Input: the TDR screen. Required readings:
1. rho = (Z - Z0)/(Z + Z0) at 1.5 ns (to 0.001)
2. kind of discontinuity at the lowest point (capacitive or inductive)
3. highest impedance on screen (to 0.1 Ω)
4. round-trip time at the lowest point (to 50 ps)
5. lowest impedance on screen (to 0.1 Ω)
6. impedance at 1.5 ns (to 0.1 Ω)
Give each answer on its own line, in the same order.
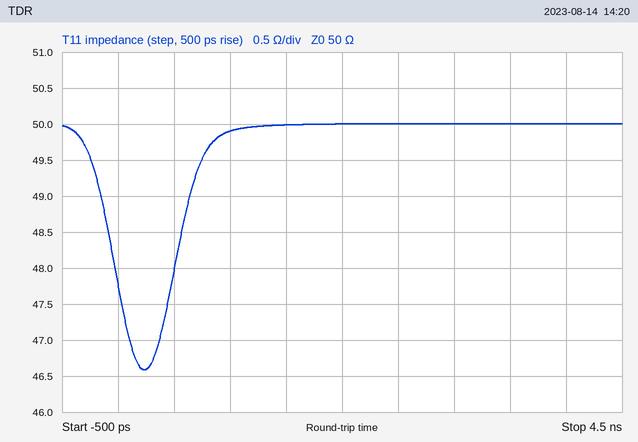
0.000
capacitive
50.0 Ω
250 ps
46.6 Ω
50.0 Ω
